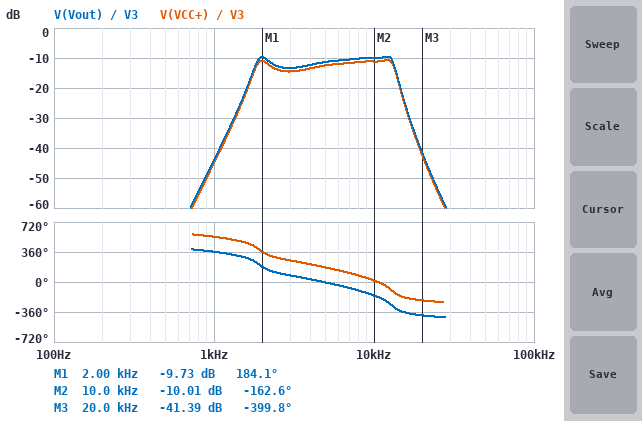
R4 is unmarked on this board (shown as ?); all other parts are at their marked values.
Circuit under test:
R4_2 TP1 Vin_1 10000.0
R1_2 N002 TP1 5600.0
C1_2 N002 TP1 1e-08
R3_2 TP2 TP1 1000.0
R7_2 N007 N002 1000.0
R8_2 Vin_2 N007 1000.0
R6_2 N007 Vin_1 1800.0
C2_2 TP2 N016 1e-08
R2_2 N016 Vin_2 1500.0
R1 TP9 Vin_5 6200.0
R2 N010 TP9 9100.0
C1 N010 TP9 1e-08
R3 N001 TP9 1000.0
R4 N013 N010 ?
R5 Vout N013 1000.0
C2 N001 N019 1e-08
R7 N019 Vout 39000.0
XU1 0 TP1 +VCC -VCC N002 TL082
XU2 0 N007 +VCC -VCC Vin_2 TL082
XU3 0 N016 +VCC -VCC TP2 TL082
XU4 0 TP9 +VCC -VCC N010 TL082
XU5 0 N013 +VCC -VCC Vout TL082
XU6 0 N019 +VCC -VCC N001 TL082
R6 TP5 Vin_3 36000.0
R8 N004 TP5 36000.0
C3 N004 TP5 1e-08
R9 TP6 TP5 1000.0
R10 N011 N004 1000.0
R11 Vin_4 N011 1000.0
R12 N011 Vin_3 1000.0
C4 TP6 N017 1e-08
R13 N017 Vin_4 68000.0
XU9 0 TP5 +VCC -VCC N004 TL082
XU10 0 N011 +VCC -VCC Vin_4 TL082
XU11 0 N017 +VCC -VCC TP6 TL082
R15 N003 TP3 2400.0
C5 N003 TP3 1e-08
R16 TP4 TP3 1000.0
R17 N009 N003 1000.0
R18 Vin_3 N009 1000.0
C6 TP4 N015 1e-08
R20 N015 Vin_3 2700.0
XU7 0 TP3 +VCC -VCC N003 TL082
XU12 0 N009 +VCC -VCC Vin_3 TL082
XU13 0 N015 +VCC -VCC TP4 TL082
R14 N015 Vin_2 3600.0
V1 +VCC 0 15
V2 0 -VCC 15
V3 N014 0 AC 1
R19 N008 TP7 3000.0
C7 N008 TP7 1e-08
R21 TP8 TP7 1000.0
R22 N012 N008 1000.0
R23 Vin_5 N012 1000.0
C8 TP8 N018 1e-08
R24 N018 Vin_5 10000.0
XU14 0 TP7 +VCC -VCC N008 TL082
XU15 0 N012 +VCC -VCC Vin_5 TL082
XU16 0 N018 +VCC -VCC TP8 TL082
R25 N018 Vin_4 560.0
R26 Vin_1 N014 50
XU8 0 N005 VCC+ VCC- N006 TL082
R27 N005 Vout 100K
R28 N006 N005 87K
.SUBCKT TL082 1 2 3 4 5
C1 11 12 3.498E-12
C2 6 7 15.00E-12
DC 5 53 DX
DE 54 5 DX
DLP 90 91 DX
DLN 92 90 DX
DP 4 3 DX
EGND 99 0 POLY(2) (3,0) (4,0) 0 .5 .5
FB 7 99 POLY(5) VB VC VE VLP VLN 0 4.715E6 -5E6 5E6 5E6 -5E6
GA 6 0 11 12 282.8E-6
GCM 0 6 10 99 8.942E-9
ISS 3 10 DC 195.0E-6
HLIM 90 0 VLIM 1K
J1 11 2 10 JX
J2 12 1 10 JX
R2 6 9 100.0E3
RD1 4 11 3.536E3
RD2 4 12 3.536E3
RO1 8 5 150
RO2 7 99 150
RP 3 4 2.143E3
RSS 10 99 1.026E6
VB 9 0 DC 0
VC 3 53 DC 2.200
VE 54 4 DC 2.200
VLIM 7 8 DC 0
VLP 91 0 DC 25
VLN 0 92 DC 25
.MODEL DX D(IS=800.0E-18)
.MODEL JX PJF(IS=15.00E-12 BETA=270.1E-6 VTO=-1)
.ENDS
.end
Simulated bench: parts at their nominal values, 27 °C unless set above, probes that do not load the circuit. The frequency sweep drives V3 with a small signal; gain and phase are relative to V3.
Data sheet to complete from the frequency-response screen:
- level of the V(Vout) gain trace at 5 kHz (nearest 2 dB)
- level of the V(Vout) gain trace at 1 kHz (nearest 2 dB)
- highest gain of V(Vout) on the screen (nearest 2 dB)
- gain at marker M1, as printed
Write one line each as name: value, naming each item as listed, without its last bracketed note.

level of the V(Vout) gain trace at 5 kHz: -12 dB
level of the V(Vout) gain trace at 1 kHz: -44 dB
highest gain of V(Vout) on the screen: -10 dB
gain at marker M1, as printed: -9.73 dB
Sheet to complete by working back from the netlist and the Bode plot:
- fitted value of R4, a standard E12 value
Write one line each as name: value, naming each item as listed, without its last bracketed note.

fitted value of R4, a standard E12 value: 3.3 kΩ
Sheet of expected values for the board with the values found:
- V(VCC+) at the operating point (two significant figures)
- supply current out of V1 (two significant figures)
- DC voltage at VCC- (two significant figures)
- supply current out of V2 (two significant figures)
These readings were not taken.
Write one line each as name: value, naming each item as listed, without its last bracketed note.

V(VCC+) at the operating point: 1.5 V
supply current out of V1: 210 mA
DC voltage at VCC-: -1.5 V
supply current out of V2: 210 mA
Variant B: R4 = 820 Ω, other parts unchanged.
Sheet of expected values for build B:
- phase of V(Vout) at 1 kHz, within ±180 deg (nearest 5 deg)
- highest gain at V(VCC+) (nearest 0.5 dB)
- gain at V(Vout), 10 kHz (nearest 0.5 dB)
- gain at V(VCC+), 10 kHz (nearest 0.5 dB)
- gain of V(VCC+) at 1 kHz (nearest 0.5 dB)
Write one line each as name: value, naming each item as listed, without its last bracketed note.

phase of V(Vout) at 1 kHz, within ±180 deg: 50 deg
highest gain at V(VCC+): 2.0 dB
gain at V(Vout), 10 kHz: 2.5 dB
gain at V(VCC+), 10 kHz: 1.5 dB
gain of V(VCC+) at 1 kHz: -44.0 dB
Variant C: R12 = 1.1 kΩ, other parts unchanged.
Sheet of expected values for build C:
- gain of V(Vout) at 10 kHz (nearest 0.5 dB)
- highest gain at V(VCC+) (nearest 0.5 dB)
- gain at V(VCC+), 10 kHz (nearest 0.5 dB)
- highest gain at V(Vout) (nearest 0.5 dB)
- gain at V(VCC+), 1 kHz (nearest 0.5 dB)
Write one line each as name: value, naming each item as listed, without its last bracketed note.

gain of V(Vout) at 10 kHz: -11.0 dB
highest gain at V(VCC+): -11.5 dB
gain at V(VCC+), 10 kHz: -12.0 dB
highest gain at V(Vout): -10.5 dB
gain at V(VCC+), 1 kHz: -46.0 dB
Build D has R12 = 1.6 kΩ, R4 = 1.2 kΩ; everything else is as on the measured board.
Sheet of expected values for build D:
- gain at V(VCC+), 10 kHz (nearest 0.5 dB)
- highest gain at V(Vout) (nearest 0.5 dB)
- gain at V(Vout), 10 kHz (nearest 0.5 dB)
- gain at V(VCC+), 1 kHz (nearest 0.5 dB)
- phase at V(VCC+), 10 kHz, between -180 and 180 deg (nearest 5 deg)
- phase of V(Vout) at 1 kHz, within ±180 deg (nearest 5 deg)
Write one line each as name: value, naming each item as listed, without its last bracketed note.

gain at V(VCC+), 10 kHz: -6.0 dB
highest gain at V(Vout): -4.0 dB
gain at V(Vout), 10 kHz: -5.0 dB
gain at V(VCC+), 1 kHz: -47.5 dB
phase at V(VCC+), 10 kHz, between -180 and 180 deg: 20 deg
phase of V(Vout) at 1 kHz, within ±180 deg: 60 deg
